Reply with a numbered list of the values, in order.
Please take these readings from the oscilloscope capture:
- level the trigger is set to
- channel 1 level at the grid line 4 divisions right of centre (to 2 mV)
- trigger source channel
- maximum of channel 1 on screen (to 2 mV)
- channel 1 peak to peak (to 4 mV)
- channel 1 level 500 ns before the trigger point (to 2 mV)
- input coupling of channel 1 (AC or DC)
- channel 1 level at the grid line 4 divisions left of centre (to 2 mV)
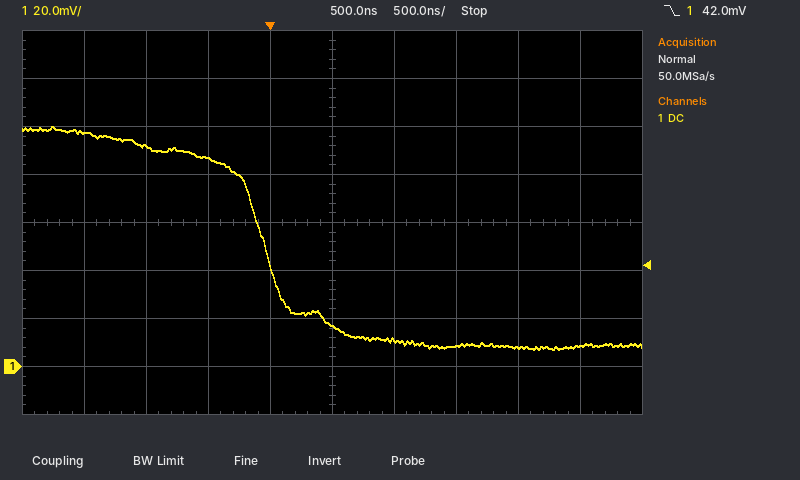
1. 42.0 mV
2. 8 mV
3. channel 1
4. 100 mV
5. 92 mV
6. 86 mV
7. DC
8. 98 mV
